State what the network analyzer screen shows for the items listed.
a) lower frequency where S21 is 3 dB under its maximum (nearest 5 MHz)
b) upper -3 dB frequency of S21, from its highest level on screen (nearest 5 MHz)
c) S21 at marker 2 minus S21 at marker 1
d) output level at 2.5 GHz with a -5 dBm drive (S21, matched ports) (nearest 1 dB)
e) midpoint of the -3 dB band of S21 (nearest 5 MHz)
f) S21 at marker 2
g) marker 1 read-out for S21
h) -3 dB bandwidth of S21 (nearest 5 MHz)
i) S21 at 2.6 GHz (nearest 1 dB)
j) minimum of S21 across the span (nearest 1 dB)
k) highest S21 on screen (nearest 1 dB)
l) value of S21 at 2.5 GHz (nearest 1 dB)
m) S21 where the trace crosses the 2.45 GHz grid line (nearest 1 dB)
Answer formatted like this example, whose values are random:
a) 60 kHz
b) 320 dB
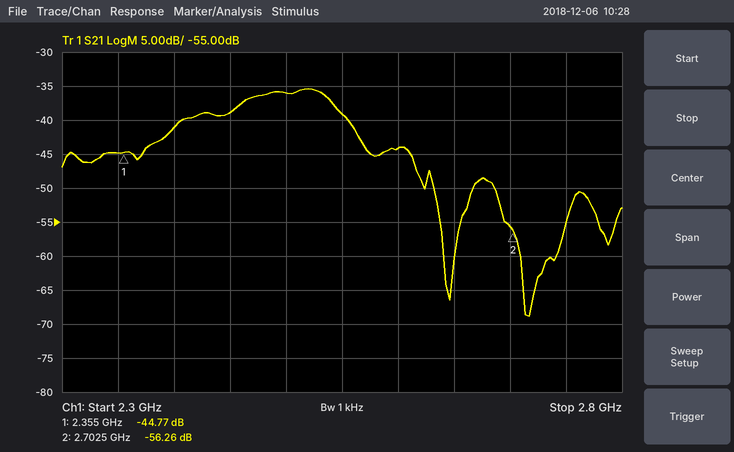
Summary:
a) 2.455 GHz
b) 2.545 GHz
c) -11.49 dB
d) -41 dBm
e) 2.500 GHz
f) -56.26 dB
g) -44.77 dB
h) 90 MHz
i) -44 dB
j) -69 dB
k) -35 dB
l) -36 dB
m) -39 dB
